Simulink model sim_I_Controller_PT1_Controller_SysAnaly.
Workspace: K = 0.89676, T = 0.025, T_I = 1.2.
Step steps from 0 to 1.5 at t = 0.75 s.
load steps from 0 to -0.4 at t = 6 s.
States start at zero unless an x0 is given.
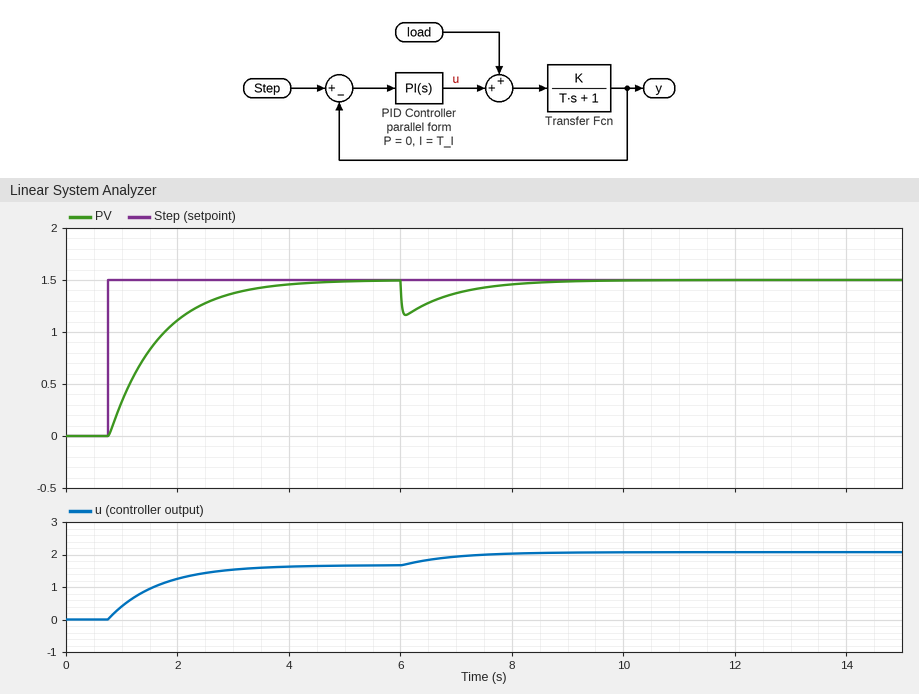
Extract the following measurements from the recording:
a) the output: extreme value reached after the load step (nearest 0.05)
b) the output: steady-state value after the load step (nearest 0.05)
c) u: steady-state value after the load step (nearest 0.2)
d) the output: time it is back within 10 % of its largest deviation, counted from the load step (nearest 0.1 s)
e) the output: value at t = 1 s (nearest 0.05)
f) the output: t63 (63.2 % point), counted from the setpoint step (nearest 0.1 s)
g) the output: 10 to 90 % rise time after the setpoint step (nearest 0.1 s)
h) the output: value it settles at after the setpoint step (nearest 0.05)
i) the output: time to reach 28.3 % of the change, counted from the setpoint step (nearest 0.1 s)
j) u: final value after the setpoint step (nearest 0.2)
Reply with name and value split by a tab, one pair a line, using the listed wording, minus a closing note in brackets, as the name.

the output: extreme value reached after the load step	1.15
the output: steady-state value after the load step	1.50
u: steady-state value after the load step	2.0
the output: time it is back within 10 % of its largest deviation, counted from the load step	2.2 s
the output: value at t = 1 s	0.35
the output: t63 (63.2 % point), counted from the setpoint step	0.9 s
the output: 10 to 90 % rise time after the setpoint step	2.0 s
the output: value it settles at after the setpoint step	1.50
the output: time to reach 28.3 % of the change, counted from the setpoint step	0.3 s
u: final value after the setpoint step	1.6
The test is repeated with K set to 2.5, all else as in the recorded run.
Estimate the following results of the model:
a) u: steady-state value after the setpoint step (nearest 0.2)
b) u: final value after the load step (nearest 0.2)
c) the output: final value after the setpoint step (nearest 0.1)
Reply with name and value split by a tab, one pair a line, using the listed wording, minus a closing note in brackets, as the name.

u: steady-state value after the setpoint step	0.6
u: final value after the load step	1.0
the output: final value after the setpoint step	1.5
